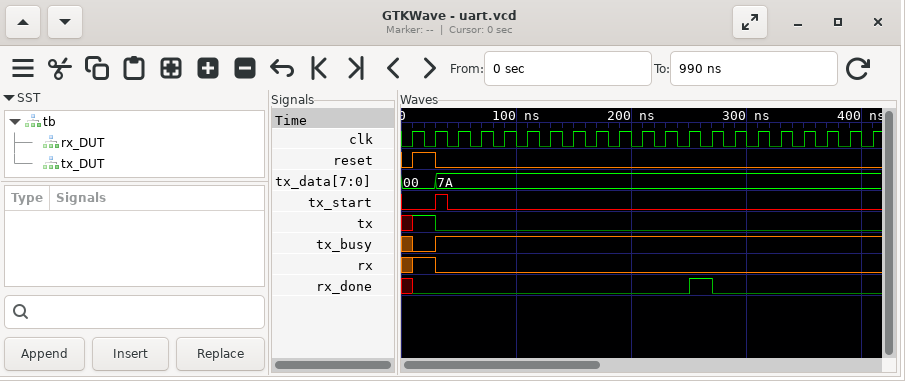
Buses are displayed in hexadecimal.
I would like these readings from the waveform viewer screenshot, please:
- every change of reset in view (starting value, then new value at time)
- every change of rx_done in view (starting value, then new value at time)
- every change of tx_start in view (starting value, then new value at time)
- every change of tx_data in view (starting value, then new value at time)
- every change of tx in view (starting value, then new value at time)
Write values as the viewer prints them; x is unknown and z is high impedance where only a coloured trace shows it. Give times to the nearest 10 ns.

0, 1 at 10 ns, 0 at 30 ns
x, 0 at 10 ns, 1 at 250 ns, 0 at 270 ns
0, 1 at 30 ns, 0 at 40 ns
00, 7A at 30 ns
x, 1 at 10 ns, 0 at 30 ns
